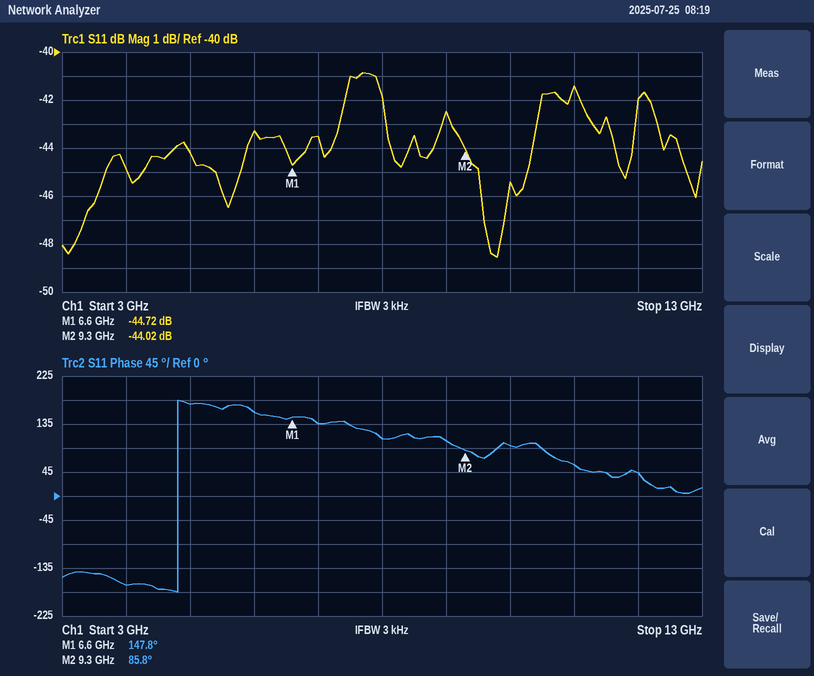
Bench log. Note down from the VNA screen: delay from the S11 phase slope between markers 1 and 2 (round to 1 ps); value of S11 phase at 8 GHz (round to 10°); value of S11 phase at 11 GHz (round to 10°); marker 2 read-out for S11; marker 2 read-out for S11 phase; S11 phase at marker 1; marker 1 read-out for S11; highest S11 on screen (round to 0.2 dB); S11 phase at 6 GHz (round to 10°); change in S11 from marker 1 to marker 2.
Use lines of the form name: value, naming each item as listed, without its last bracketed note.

delay from the S11 phase slope between markers 1 and 2: 64 ps
value of S11 phase at 8 GHz: 110°
value of S11 phase at 11 GHz: 60°
marker 2 read-out for S11: -44.02 dB
marker 2 read-out for S11 phase: 85.8°
S11 phase at marker 1: 147.8°
marker 1 read-out for S11: -44.72 dB
highest S11 on screen: -40.8 dB
S11 phase at 6 GHz: 160°
change in S11 from marker 1 to marker 2: 0.70 dB
